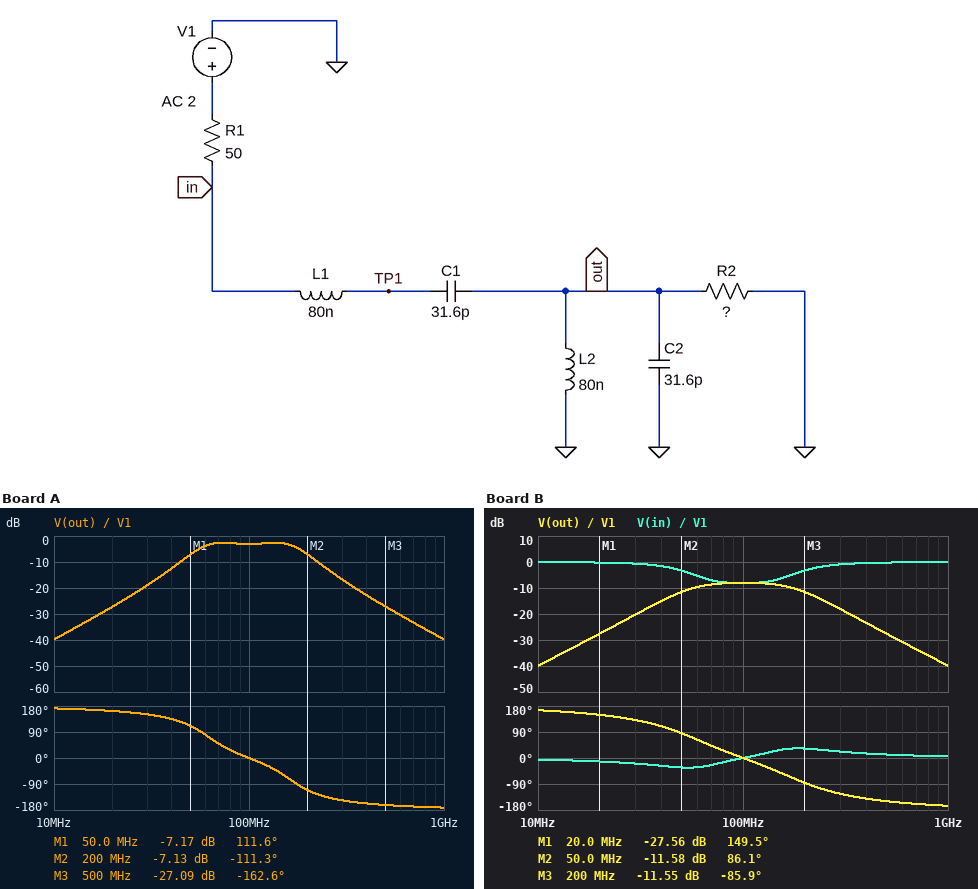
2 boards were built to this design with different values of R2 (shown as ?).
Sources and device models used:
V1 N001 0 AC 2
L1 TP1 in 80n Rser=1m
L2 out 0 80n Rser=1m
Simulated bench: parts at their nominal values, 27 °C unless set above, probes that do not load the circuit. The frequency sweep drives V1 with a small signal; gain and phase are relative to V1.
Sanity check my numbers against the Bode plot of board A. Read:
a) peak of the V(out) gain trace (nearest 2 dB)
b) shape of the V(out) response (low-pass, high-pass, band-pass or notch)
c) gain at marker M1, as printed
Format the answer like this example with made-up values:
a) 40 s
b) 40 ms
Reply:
a) -2 dB
b) band-pass
c) -7.17 dB
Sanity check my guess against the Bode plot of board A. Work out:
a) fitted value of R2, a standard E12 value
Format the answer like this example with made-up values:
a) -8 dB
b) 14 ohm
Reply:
a) 120 Ω
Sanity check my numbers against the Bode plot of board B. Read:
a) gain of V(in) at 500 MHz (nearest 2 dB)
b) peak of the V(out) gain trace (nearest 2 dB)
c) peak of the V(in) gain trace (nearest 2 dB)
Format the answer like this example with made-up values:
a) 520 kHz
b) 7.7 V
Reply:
a) 0 dB
b) -8 dB
c) 0 dB
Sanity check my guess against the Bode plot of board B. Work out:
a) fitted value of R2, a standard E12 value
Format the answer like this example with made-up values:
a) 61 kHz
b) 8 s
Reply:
a) 33 Ω
